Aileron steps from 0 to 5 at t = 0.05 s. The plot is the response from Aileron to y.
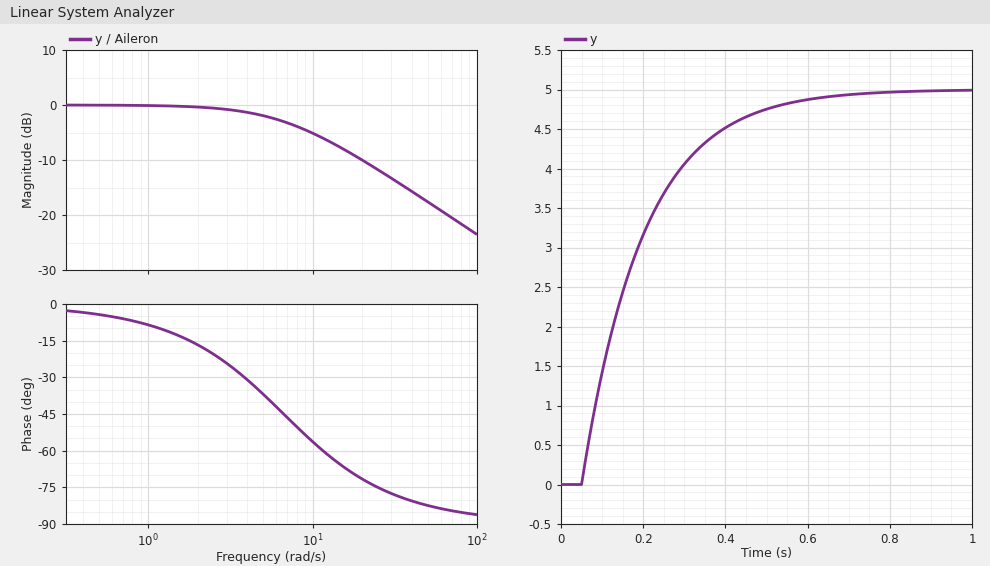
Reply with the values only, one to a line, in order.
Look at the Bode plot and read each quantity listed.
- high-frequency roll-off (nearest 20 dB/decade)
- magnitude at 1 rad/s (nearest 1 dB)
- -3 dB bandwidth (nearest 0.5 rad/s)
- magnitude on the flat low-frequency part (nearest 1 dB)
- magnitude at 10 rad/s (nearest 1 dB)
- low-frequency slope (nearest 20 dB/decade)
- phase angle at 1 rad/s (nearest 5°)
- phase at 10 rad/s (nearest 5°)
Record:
-20 dB/decade
0 dB
6.5 rad/s
0 dB
-5 dB
0 dB/decade
-10°
-55°
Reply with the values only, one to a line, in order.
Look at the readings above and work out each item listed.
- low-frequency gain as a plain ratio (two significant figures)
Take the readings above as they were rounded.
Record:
1.0
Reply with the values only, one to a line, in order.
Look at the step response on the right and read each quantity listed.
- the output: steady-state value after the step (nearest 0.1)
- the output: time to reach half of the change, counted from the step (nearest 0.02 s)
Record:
5.0
0.10 s
